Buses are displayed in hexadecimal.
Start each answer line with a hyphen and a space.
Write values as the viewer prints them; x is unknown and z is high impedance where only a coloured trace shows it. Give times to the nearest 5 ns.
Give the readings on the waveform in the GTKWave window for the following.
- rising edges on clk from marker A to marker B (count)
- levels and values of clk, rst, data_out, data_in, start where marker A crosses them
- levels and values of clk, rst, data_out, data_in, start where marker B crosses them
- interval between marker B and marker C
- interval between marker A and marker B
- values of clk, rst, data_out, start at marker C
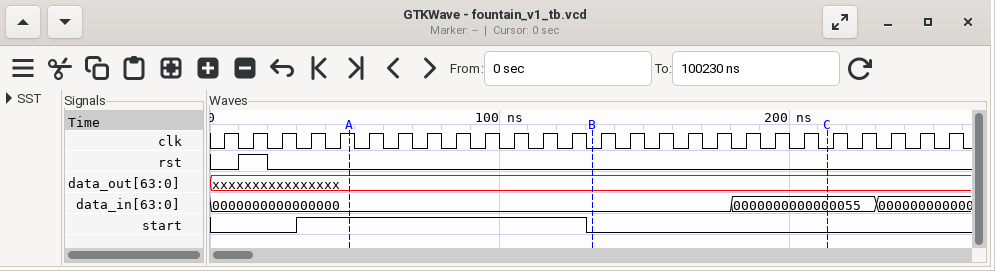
- 8
- clk=1, rst=0, data_out=xxxxxxxxxxxxxxxx, data_in=0000000000000000, start=1
- clk=0, rst=0, data_out=xxxxxxxxxxxxxxxx, data_in=0000000000000000, start=0
- 80 ns
- 85 ns
- clk=0, rst=0, data_out=xxxxxxxxxxxxxxxx, start=0
